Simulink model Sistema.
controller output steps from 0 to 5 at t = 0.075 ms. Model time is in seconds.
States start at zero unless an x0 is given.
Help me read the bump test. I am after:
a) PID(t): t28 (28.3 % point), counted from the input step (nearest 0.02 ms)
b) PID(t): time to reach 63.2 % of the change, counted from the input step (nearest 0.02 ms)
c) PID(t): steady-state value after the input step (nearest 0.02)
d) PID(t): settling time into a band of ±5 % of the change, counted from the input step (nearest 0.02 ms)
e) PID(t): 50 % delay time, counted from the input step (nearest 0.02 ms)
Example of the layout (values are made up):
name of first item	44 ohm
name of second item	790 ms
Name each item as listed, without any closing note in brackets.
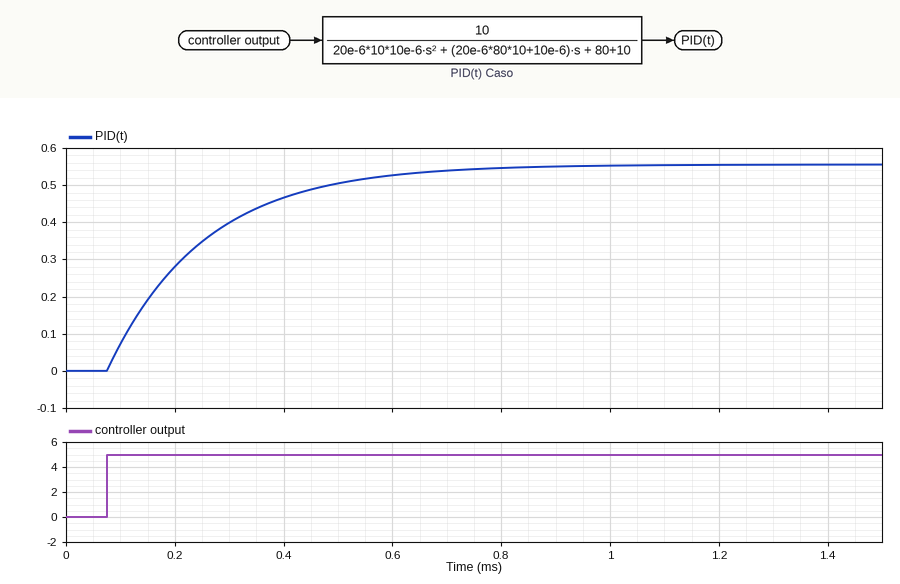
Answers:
PID(t): t28 (28.3 % point), counted from the input step	0.06 ms
PID(t): time to reach 63.2 % of the change, counted from the input step	0.18 ms
PID(t): steady-state value after the input step	0.56
PID(t): settling time into a band of ±5 % of the change, counted from the input step	0.54 ms
PID(t): 50 % delay time, counted from the input step	0.12 ms
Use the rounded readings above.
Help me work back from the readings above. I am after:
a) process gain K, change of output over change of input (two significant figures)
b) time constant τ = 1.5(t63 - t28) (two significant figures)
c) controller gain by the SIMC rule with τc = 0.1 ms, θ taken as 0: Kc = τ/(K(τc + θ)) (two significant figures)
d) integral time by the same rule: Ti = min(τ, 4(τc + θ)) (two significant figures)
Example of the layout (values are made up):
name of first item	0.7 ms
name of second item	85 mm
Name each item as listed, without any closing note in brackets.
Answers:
process gain K, change of output over change of input	0.11
time constant τ = 1.5(t63 - t28)	0.18 ms
controller gain by the SIMC rule with τc = 0.1 ms, θ taken as 0: Kc = τ/(K(τc + θ))	16
integral time by the same rule: Ti = min(τ, 4(τc + θ))	0.18 ms
